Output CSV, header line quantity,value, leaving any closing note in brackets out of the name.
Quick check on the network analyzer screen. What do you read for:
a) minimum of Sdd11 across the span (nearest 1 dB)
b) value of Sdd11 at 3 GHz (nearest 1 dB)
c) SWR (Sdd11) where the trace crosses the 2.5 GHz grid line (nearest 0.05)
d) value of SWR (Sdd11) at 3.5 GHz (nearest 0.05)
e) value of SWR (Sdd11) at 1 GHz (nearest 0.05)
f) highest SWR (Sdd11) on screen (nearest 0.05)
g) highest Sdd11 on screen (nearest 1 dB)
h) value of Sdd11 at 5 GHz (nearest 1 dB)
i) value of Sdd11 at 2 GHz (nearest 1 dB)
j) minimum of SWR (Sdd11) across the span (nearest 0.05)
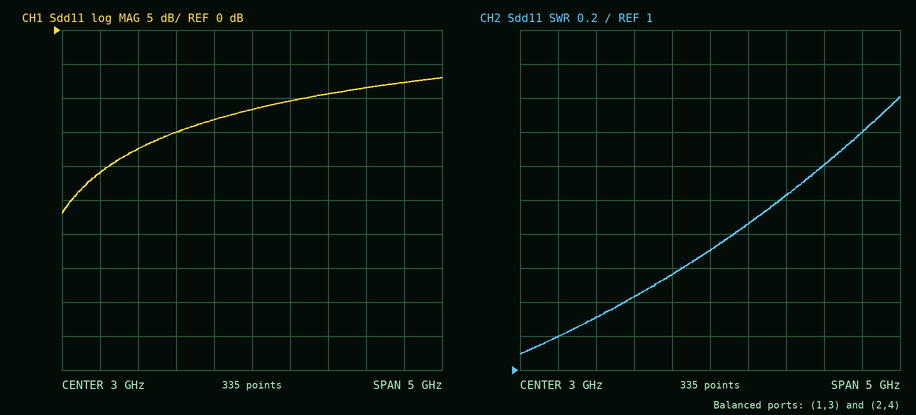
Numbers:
quantity,value
minimum of Sdd11 across the span,-27 dB
value of Sdd11 at 3 GHz,-12 dB
SWR (Sdd11) where the trace crosses the 2.5 GHz grid line,1.55
value of SWR (Sdd11) at 3.5 GHz,1.85
value of SWR (Sdd11) at 1 GHz,1.20
highest SWR (Sdd11) on screen,2.60
highest Sdd11 on screen,-7 dB
value of Sdd11 at 5 GHz,-8 dB
value of Sdd11 at 2 GHz,-15 dB
minimum of SWR (Sdd11) across the span,1.10
